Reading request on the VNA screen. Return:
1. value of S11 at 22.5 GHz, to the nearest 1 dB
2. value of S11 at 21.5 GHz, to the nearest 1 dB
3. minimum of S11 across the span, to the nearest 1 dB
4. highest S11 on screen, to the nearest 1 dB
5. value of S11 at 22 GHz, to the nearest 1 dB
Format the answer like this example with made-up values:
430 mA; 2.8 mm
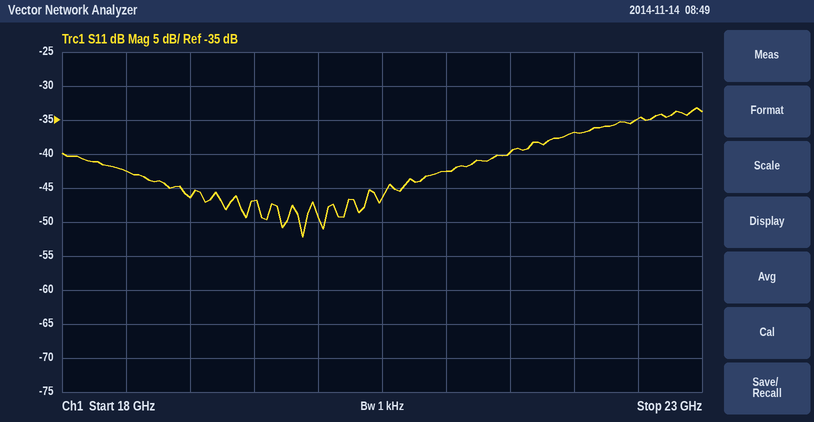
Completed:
-35 dB; -40 dB; -52 dB; -33 dB; -37 dB
